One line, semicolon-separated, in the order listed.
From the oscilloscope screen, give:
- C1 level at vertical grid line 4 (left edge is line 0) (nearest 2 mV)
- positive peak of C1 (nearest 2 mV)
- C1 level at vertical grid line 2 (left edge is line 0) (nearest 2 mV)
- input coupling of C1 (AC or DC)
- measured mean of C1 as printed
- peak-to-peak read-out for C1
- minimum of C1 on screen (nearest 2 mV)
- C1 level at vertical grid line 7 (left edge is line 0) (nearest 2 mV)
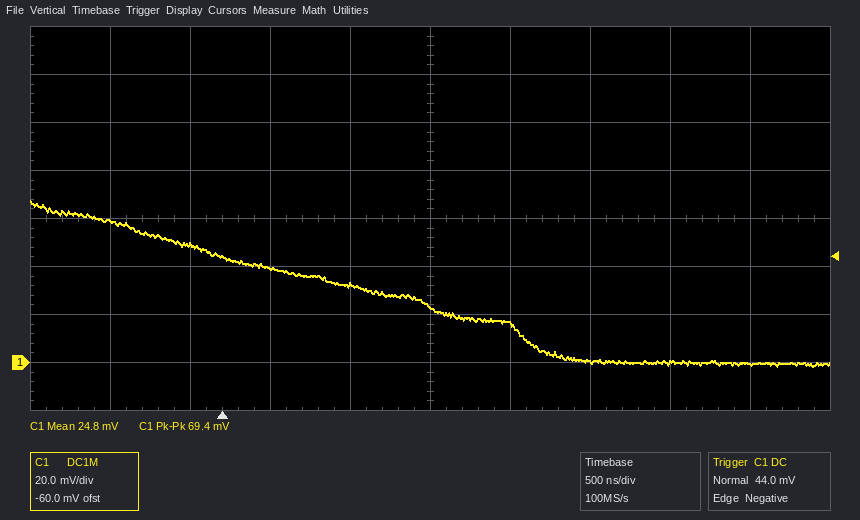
32 mV; 68 mV; 50 mV; DC; 24.8 mV; 69.4 mV; -2 mV; 0 mV
